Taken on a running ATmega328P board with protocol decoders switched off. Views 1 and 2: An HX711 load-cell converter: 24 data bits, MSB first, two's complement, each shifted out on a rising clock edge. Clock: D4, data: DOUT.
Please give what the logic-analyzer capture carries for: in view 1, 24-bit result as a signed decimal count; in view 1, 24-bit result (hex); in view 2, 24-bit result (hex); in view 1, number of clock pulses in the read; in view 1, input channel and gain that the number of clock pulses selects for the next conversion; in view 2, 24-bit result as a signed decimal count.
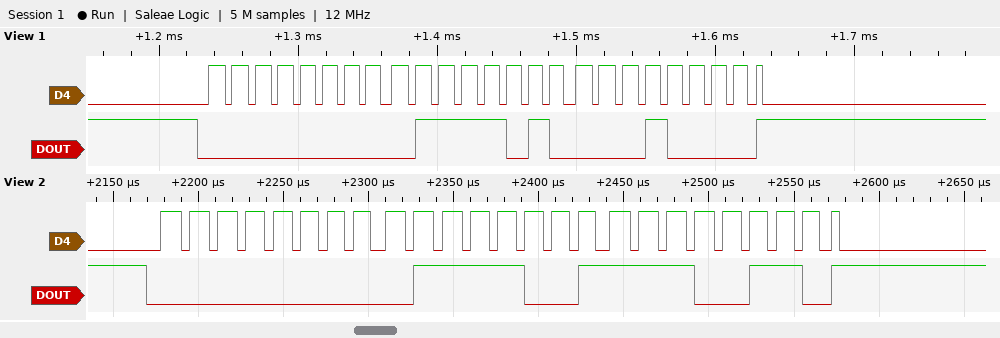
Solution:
31248
0x007A10
0x0079E6
25
channel A, gain 128
31206
